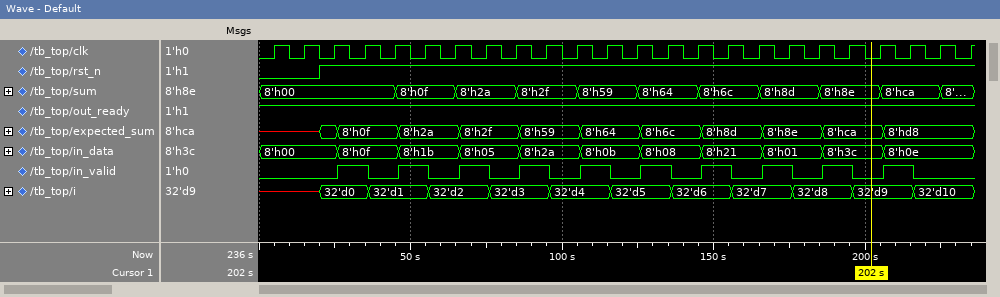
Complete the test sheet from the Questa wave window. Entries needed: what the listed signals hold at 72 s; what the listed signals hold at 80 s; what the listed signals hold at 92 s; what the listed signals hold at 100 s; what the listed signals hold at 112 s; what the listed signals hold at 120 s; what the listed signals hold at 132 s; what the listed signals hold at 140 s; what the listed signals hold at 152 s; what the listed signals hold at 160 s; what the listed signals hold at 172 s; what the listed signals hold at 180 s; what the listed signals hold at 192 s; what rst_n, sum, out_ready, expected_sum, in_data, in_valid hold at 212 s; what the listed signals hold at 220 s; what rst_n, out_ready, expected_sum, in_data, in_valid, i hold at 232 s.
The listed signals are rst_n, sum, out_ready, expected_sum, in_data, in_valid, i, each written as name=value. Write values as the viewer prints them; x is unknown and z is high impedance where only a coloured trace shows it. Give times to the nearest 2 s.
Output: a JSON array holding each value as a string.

["rst_n=1, sum=8'h2a, out_ready=1, expected_sum=8'h2f, in_data=8'h05, in_valid=1, i=32'd2", "rst_n=1, sum=8'h2a, out_ready=1, expected_sum=8'h2f, in_data=8'h05, in_valid=0, i=32'd3", "rst_n=1, sum=8'h2f, out_ready=1, expected_sum=8'h59, in_data=8'h2a, in_valid=1, i=32'd3", "rst_n=1, sum=8'h2f, out_ready=1, expected_sum=8'h59, in_data=8'h2a, in_valid=0, i=32'd4", "rst_n=1, sum=8'h59, out_ready=1, expected_sum=8'h64, in_data=8'h0b, in_valid=1, i=32'd4", "rst_n=1, sum=8'h59, out_ready=1, expected_sum=8'h64, in_data=8'h0b, in_valid=0, i=32'd5", "rst_n=1, sum=8'h64, out_ready=1, expected_sum=8'h6c, in_data=8'h08, in_valid=1, i=32'd5", "rst_n=1, sum=8'h64, out_ready=1, expected_sum=8'h6c, in_data=8'h08, in_valid=0, i=32'd6", "rst_n=1, sum=8'h6c, out_ready=1, expected_sum=8'h8d, in_data=8'h21, in_valid=1, i=32'd6", "rst_n=1, sum=8'h6c, out_ready=1, expected_sum=8'h8d, in_data=8'h21, in_valid=0, i=32'd7", "rst_n=1, sum=8'h8d, out_ready=1, expected_sum=8'h8e, in_data=8'h01, in_valid=1, i=32'd7", "rst_n=1, sum=8'h8d, out_ready=1, expected_sum=8'h8e, in_data=8'h01, in_valid=0, i=32'd8", "rst_n=1, sum=8'h8e, out_ready=1, expected_sum=8'hca, in_data=8'h3c, in_valid=1, i=32'd8", "rst_n=1, sum=8'hca, out_ready=1, expected_sum=8'hd8, in_data=8'h0e, in_valid=1", "rst_n=1, sum=8'hca, out_ready=1, expected_sum=8'hd8, in_data=8'h0e, in_valid=0, i=32'd10", "rst_n=1, out_ready=1, expected_sum=8'hd8, in_data=8'h0e, in_valid=0, i=32'd10"]
